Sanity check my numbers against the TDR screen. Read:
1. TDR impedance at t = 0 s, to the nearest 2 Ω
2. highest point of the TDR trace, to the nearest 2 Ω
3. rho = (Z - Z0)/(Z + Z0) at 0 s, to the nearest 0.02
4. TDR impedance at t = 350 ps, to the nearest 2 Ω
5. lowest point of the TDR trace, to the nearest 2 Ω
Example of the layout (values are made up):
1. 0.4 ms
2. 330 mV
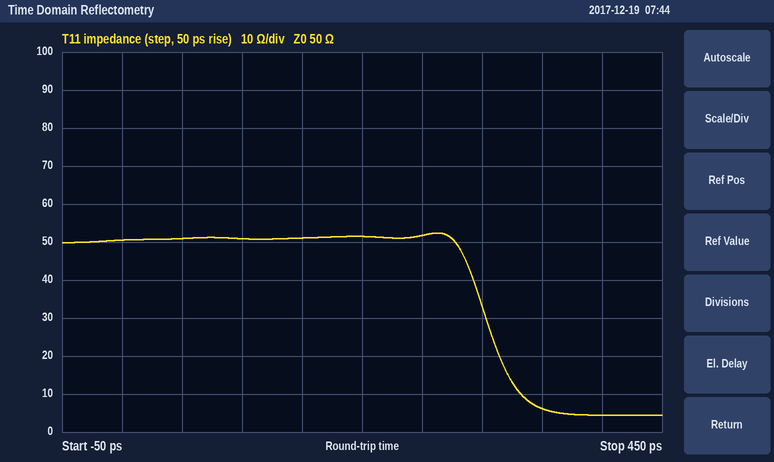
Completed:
1. 50 Ω
2. 52 Ω
3. 0.00
4. 6 Ω
5. 4 Ω
